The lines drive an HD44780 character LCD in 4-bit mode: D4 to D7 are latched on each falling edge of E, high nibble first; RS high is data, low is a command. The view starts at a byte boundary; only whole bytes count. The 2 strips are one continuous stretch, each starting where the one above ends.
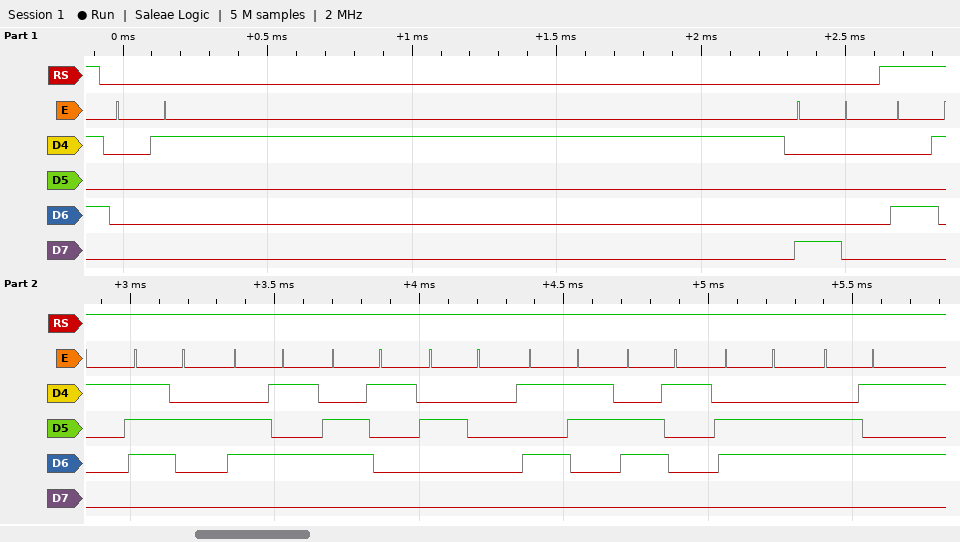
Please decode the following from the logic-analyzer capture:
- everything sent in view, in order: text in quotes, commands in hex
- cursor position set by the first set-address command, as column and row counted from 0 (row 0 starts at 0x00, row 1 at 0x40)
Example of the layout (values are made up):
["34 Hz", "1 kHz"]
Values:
["0x01 0x80 \"Area Safe\"", "column 0, row 0"]
